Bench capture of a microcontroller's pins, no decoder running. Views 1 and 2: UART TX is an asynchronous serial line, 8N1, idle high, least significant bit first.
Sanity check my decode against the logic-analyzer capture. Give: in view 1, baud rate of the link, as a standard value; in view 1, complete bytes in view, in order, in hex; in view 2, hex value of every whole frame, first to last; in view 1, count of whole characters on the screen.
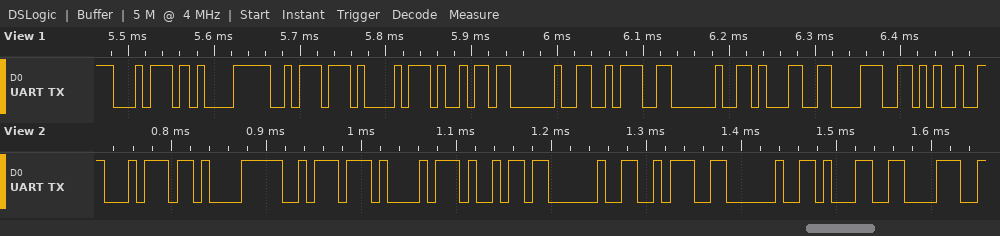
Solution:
115200 baud
74 E1 BA A1 69 20 3A 20 31 38 25
0x74 0xE1 0xBA 0xA1 0x69 0x20 0x3A 0x20 0x31 0x38
11
